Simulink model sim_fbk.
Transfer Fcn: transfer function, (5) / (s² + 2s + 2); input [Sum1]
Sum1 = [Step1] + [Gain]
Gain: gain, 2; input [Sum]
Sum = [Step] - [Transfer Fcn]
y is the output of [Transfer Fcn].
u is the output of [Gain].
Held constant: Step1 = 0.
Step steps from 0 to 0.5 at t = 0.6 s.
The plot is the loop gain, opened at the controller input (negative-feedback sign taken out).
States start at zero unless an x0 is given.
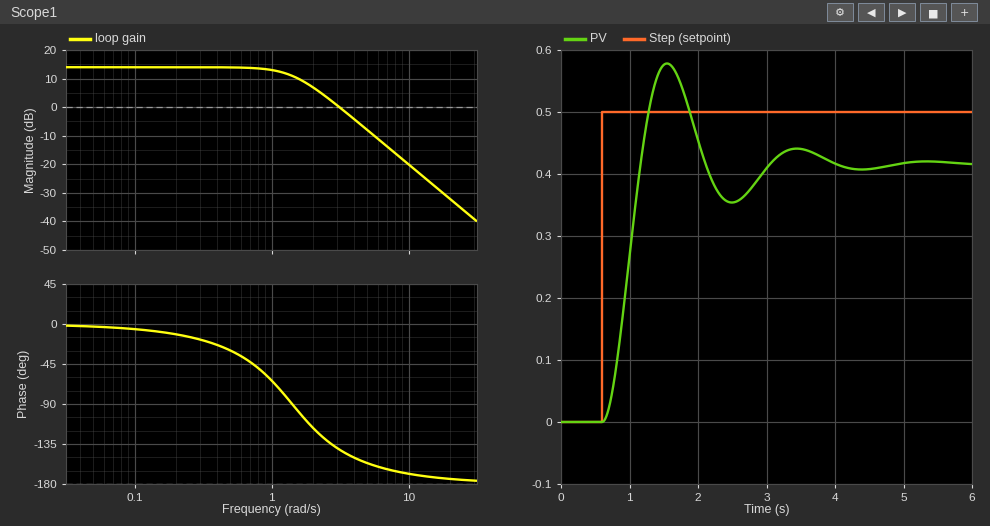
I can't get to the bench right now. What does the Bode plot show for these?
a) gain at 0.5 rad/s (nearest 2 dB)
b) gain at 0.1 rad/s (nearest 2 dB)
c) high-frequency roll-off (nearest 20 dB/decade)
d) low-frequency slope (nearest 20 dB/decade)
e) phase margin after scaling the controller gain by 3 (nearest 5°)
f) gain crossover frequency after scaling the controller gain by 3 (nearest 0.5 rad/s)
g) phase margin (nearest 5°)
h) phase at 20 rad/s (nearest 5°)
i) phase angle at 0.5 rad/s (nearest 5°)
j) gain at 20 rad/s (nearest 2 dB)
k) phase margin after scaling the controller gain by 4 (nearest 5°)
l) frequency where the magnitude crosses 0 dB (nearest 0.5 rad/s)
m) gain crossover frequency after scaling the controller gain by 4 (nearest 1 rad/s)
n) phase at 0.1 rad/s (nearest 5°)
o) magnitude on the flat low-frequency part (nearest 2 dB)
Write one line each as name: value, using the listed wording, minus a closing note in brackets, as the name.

gain at 0.5 rad/s: 14 dB
gain at 0.1 rad/s: 14 dB
high-frequency roll-off: -40 dB/decade
low-frequency slope: 0 dB/decade
phase margin after scaling the controller gain by 3: 20°
gain crossover frequency after scaling the controller gain by 3: 5.5 rad/s
phase margin: 40°
phase at 20 rad/s: -175°
phase angle at 0.5 rad/s: -30°
gain at 20 rad/s: -32 dB
phase margin after scaling the controller gain by 4: 20°
frequency where the magnitude crosses 0 dB: 3.0 rad/s
gain crossover frequency after scaling the controller gain by 4: 6 rad/s
phase at 0.1 rad/s: -5°
magnitude on the flat low-frequency part: 14 dB
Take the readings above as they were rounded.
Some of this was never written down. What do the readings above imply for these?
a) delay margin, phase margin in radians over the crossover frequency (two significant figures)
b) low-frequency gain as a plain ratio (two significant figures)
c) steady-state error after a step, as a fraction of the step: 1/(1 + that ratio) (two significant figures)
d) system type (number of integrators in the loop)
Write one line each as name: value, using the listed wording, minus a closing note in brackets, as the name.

delay margin, phase margin in radians over the crossover frequency: 0.23 s
low-frequency gain as a plain ratio: 5.0
steady-state error after a step, as a fraction of the step: 1/(1 + that ratio): 0.17
system type: 0
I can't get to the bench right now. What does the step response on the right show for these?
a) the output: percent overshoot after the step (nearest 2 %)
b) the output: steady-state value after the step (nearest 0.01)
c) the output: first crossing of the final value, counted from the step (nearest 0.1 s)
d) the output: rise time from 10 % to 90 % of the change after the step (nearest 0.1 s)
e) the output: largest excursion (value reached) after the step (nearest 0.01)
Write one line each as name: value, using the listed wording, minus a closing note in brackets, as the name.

the output: percent overshoot after the step: 38 %
the output: steady-state value after the step: 0.42
the output: first crossing of the final value, counted from the step: 0.6 s
the output: rise time from 10 % to 90 % of the change after the step: 0.4 s
the output: largest excursion (value reached) after the step: 0.58
